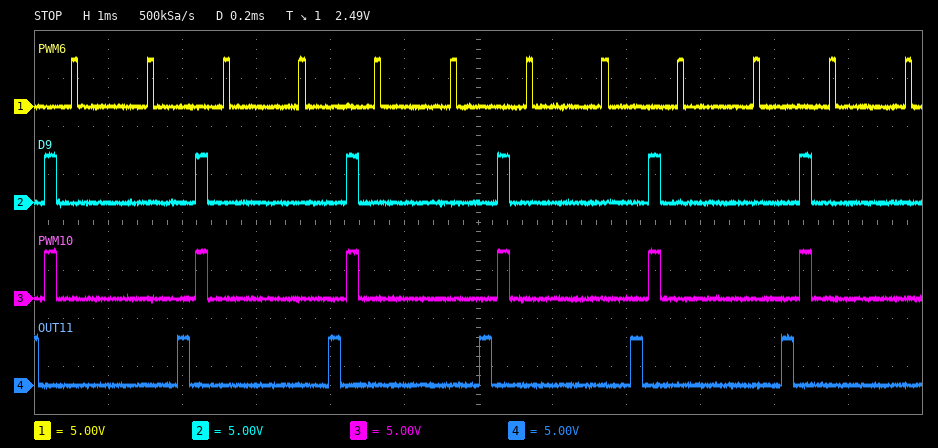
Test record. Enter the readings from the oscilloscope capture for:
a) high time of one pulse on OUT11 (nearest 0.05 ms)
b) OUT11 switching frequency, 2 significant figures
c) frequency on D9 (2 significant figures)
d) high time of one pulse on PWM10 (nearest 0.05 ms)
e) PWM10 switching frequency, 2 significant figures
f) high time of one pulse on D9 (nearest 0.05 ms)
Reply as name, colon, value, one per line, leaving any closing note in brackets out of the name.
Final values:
high time of one pulse on OUT11: 0.15 ms
OUT11 switching frequency, 2 significant figures: 490 Hz
frequency on D9: 490 Hz
high time of one pulse on PWM10: 0.15 ms
PWM10 switching frequency, 2 significant figures: 490 Hz
high time of one pulse on D9: 0.15 ms
